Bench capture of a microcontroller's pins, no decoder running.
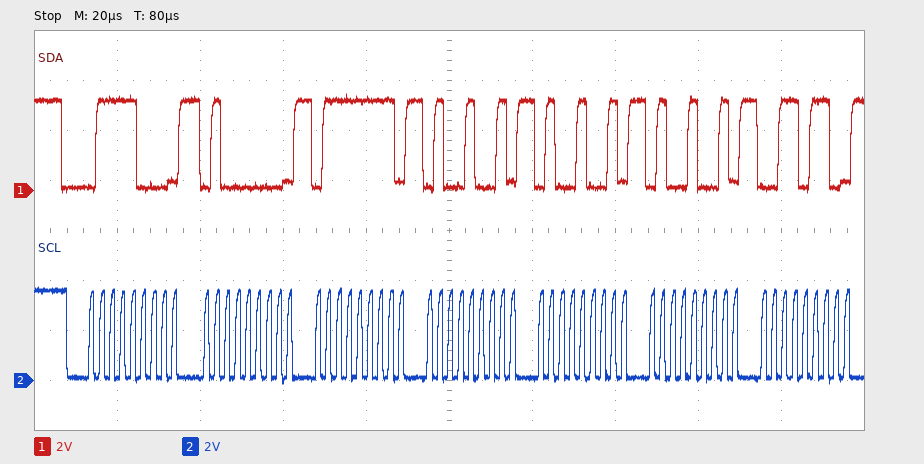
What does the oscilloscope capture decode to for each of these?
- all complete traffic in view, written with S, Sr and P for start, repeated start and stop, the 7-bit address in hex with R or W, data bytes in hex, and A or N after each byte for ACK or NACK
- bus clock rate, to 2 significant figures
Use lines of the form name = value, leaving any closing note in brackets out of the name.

all complete traffic in view, written with S, Sr and P for start, repeated start and stop, the 7-bit address in hex with R or W, data bytes in hex, and A or N after each byte for ACK or NACK = S 3CW A 40 A 7F A 49 A 49 A 49 A 36 A
bus clock rate, to 2 significant figures = 400 kHz
